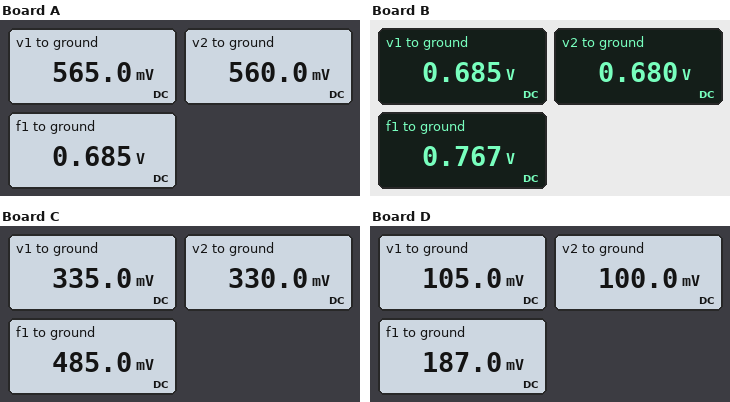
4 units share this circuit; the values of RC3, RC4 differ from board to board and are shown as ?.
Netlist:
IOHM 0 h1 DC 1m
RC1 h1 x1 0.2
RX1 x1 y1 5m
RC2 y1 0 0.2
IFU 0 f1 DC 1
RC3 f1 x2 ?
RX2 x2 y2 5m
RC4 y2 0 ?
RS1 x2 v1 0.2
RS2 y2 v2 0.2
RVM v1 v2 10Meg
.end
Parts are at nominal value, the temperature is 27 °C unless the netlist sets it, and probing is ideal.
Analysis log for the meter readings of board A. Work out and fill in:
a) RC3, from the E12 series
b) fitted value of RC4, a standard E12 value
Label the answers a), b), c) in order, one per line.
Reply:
a) 0.12 Ω
b) 0.56 Ω
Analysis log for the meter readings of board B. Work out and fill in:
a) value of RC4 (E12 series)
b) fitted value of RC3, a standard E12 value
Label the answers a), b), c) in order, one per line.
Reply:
a) 0.68 Ω
b) 0.082 Ω
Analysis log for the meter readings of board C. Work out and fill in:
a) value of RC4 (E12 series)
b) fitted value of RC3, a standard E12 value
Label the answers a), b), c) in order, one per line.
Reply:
a) 0.33 Ω
b) 0.15 Ω
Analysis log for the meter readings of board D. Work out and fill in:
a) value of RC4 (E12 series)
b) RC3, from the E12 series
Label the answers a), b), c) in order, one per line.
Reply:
a) 0.1 Ω
b) 0.082 Ω
